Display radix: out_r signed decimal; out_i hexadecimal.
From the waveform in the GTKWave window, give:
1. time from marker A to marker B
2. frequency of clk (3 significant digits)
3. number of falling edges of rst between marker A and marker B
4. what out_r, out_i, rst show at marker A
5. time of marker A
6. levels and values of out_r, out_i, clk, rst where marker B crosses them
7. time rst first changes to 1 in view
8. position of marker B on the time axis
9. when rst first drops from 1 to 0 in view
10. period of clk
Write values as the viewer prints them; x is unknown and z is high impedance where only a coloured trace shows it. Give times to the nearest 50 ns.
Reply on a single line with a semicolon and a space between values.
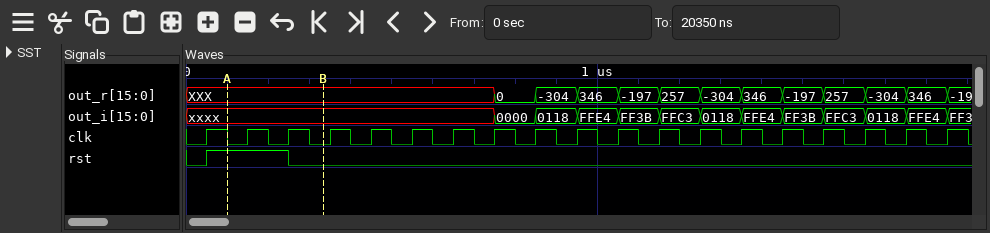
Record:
250 ns; 10.0 MHz; 1; out_r=XXX, out_i=xxxx, rst=1; 100 ns; out_r=XXX, out_i=xxxx, clk=0, rst=0; 50 ns; 350 ns; 250 ns; 100 ns
